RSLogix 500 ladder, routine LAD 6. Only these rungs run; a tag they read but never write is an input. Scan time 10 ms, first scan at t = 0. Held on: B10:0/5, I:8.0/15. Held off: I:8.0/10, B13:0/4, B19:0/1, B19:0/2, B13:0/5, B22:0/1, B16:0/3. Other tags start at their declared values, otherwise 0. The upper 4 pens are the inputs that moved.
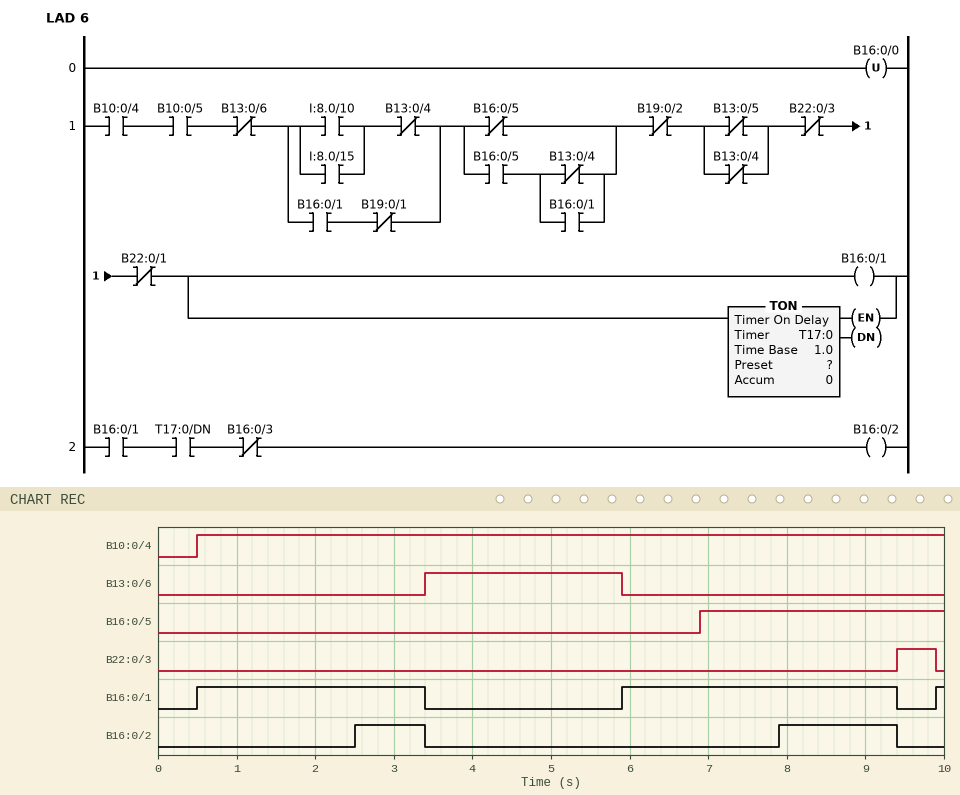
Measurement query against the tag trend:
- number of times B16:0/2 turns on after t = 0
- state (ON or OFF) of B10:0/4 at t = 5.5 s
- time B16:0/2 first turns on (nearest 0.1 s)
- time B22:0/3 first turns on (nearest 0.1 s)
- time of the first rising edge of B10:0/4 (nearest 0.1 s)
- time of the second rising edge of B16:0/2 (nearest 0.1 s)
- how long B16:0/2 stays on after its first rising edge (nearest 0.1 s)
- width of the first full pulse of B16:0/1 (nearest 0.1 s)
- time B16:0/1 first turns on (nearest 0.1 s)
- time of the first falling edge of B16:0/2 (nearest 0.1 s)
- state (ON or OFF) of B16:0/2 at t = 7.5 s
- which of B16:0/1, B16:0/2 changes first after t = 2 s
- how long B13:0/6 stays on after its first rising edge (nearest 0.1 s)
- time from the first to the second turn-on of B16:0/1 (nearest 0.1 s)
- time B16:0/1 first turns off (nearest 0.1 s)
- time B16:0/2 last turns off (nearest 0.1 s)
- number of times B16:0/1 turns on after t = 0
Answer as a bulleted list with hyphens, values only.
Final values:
- 2
- ON
- 2.5 s
- 9.4 s
- 0.5 s
- 7.9 s
- 0.9 s
- 2.9 s
- 0.5 s
- 3.4 s
- OFF
- B16:0/2
- 2.5 s
- 5.4 s
- 3.4 s
- 9.4 s
- 3
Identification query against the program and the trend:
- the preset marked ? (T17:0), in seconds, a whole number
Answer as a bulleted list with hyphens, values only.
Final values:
- 2 s
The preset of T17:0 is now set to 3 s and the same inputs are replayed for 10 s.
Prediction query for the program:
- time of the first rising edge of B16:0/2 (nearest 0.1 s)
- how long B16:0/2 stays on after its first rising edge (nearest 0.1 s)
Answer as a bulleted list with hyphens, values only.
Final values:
- 8.9 s
- 0.5 s
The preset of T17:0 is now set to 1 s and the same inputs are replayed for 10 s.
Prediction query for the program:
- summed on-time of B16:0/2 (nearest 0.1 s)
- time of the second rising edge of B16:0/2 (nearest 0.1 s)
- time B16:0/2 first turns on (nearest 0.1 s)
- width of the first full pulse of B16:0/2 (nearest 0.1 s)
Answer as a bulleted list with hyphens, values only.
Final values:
- 4.4 s
- 6.9 s
- 1.5 s
- 1.9 s
